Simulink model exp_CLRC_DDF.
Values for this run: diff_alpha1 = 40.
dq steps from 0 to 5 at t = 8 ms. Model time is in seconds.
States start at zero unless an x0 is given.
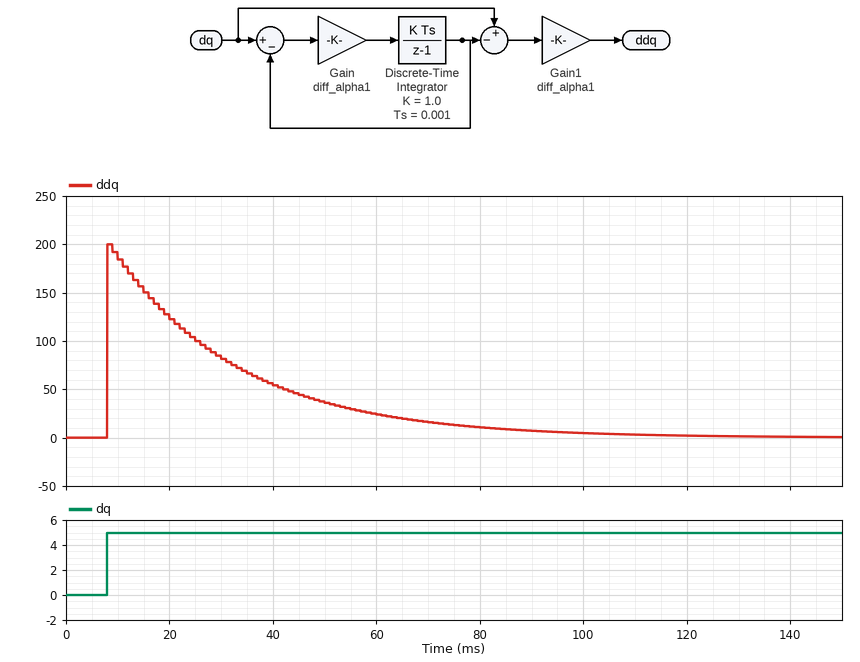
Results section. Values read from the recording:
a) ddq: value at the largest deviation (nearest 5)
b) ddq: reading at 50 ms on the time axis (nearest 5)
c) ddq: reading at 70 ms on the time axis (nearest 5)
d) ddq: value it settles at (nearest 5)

200
35
15
0
